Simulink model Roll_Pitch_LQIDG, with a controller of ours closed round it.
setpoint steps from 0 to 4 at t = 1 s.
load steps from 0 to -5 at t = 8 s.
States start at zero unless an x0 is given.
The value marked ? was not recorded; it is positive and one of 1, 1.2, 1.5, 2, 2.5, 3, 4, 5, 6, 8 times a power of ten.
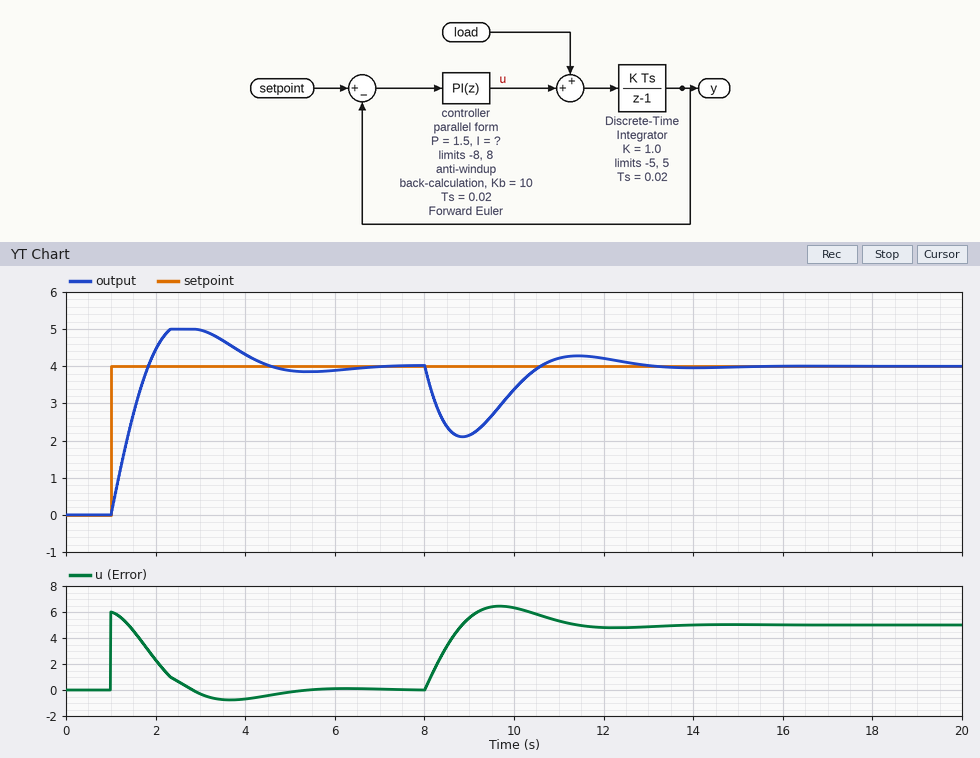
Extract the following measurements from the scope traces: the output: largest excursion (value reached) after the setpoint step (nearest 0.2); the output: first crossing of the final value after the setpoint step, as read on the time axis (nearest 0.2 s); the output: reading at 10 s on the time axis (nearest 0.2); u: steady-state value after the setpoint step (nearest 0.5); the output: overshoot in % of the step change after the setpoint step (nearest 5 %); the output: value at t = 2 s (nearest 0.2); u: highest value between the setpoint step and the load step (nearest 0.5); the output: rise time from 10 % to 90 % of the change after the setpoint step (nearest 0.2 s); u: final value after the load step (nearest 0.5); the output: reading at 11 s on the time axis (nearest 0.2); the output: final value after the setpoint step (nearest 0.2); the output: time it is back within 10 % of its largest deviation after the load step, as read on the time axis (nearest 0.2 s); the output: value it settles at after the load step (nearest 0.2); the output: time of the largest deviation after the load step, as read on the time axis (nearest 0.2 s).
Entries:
5.0
1.8 s
3.4
0.0
25 %
4.4
6.0
0.6 s
5.0
4.2
4.0
12.2 s
4.0
8.8 s
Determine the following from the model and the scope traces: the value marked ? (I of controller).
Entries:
2
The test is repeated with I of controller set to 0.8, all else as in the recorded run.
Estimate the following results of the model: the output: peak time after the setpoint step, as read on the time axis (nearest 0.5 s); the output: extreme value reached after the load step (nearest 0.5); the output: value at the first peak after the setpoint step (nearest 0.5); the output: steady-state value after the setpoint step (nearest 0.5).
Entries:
3.5 s
1.5
4.5
4.0
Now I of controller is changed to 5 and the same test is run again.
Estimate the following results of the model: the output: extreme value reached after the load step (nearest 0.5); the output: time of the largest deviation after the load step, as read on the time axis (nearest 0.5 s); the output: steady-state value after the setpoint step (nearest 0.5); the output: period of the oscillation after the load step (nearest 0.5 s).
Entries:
2.5
8.5 s
4.0
3.0 s
